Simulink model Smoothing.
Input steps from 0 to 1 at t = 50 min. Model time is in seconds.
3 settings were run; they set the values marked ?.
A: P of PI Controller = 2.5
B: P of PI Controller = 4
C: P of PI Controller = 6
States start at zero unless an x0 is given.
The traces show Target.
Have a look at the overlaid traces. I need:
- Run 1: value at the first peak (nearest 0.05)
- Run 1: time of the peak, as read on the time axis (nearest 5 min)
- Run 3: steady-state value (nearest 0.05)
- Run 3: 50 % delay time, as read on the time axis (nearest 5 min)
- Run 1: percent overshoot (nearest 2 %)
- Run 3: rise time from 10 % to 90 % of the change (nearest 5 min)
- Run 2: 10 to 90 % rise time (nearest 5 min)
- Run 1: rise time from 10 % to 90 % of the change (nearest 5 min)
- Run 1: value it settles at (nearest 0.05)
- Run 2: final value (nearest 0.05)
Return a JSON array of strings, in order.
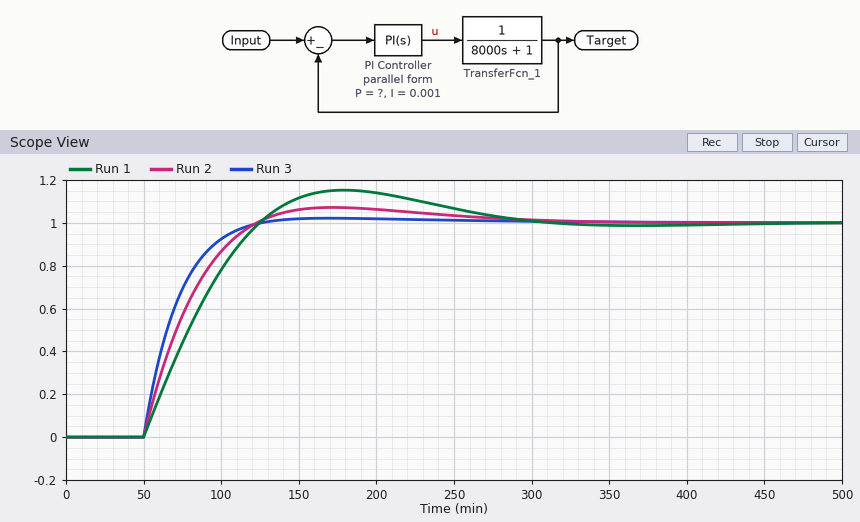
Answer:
["1.15", "180 min", "1.00", "65 min", "16 %", "45 min", "50 min", "55 min", "1.00", "1.00"]
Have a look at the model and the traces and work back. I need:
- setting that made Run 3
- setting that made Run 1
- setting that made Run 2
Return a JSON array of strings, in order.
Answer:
["C", "A", "B"]
